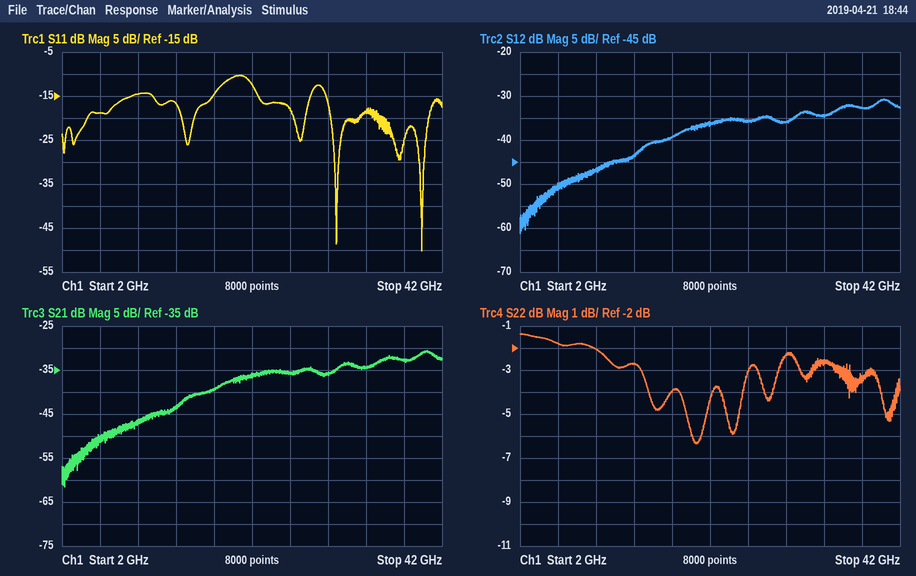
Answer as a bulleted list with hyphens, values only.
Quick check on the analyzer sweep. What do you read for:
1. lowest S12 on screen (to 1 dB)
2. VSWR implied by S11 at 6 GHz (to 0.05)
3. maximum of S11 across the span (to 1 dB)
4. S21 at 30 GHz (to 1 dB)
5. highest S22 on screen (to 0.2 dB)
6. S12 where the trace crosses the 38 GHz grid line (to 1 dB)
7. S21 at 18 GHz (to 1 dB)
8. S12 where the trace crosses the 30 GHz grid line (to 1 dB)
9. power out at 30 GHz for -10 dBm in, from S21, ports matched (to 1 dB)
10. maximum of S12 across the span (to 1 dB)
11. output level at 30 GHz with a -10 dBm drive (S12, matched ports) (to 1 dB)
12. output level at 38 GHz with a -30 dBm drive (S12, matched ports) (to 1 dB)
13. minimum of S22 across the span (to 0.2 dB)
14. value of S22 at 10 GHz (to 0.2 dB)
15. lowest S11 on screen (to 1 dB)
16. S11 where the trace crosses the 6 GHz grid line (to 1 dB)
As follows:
- -61 dB
- 1.25
- -10 dB
- -36 dB
- -1.4 dB
- -33 dB
- -39 dB
- -36 dB
- -46 dBm
- -31 dB
- -46 dBm
- -63 dBm
- -6.4 dB
- -2.0 dB
- -50 dB
- -19 dB
